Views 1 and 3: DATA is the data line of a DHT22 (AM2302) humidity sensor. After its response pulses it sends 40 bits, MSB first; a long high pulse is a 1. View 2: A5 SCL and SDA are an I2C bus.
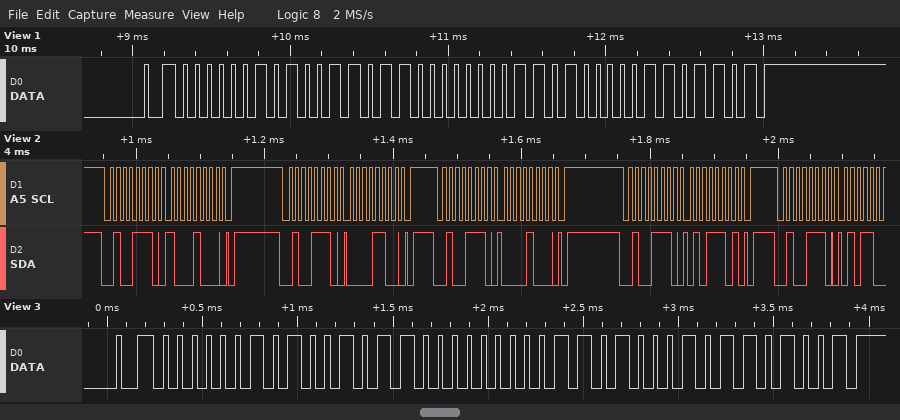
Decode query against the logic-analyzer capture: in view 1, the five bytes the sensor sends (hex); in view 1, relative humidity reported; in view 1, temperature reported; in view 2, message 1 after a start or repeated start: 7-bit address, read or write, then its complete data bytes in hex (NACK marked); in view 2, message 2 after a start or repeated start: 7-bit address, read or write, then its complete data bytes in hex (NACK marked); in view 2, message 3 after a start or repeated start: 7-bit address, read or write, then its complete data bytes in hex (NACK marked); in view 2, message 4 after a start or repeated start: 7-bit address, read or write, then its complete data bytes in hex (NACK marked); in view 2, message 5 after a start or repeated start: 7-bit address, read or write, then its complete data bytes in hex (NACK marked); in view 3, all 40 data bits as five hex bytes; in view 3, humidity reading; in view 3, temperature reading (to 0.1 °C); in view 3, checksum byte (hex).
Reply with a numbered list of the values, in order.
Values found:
1. 02 9B 00 D0 6D
2. 66.7 %
3. 20.8 °C
4. 0x27 write: 88
5. 0x27 write: 0C
6. 0x27 write: 08
7. 0x27 write: 5D
8. 0x27 write
9. 02 96 00 D1 69
10. 66.2 %
11. 20.9 °C
12. 0x69
